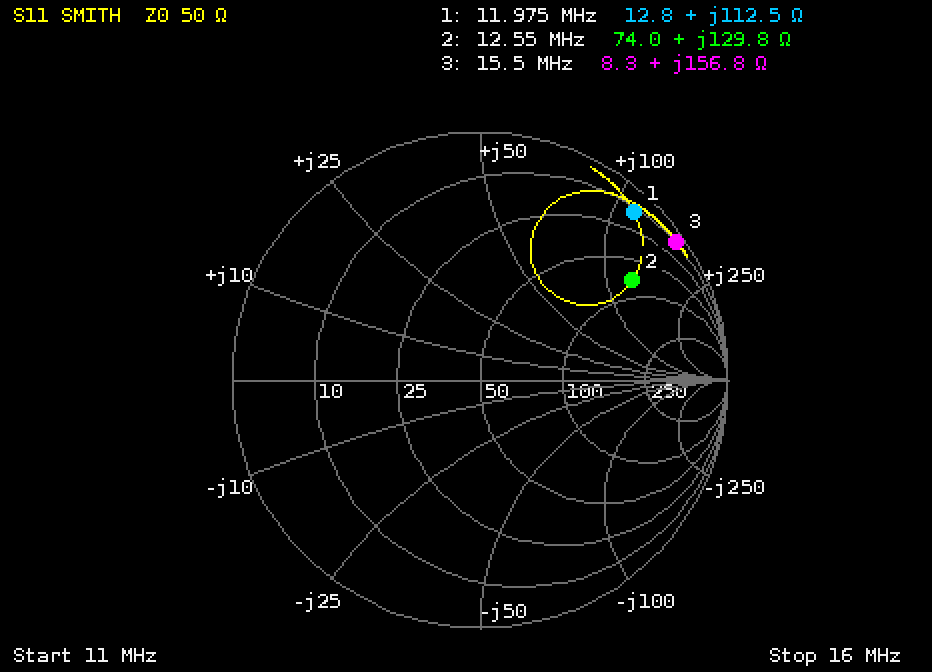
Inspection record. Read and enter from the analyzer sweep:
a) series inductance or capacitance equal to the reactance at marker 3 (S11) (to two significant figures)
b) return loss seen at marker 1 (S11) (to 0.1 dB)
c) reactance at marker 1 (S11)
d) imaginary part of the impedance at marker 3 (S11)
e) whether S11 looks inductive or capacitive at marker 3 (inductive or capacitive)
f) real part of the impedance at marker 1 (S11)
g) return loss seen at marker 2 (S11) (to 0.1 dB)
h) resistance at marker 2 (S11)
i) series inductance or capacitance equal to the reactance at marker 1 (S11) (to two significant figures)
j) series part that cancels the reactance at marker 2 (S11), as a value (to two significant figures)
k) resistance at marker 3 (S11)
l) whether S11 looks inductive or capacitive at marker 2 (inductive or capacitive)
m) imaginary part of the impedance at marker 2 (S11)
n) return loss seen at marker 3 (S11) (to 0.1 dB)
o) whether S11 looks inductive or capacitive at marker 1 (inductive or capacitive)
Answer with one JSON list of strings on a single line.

["1.6 µH", "0.7 dB", "+112.5 Ω", "+156.8 Ω", "inductive", "12.8 Ω", "2.7 dB", "74.0 Ω", "1.5 µH", "98 pF", "8.3 Ω", "inductive", "+129.8 Ω", "0.3 dB", "inductive"]
